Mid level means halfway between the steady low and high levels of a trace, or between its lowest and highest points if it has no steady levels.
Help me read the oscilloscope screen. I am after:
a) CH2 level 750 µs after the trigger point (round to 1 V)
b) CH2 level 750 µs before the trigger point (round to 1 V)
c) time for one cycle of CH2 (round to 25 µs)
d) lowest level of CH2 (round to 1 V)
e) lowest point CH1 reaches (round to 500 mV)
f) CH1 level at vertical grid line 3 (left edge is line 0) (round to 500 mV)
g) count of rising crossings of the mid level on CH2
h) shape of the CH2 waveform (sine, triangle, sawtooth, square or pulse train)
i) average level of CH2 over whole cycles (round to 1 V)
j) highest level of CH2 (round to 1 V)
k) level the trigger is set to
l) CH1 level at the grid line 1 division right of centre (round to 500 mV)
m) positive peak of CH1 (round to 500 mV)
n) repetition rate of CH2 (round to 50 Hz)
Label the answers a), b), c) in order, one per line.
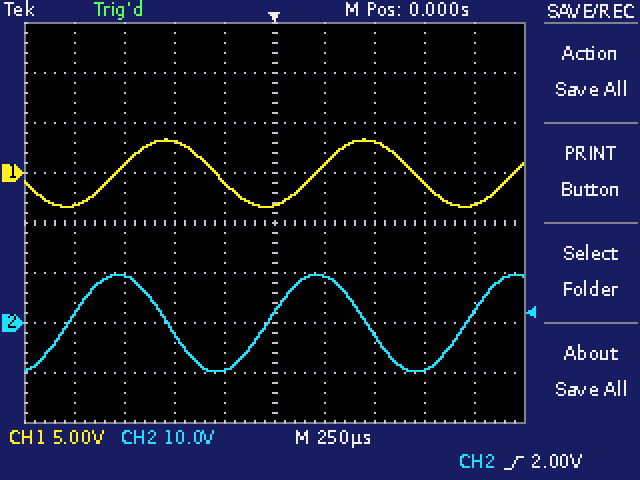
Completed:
a) -9 V
b) 9 V
c) 1.000 ms
d) -10 V
e) -3.5 V
f) 3.0 V
g) 3
h) sine
i) 0 V
j) 10 V
k) 2.00 V
l) 1.0 V
m) 3.5 V
n) 1.00 kHz
